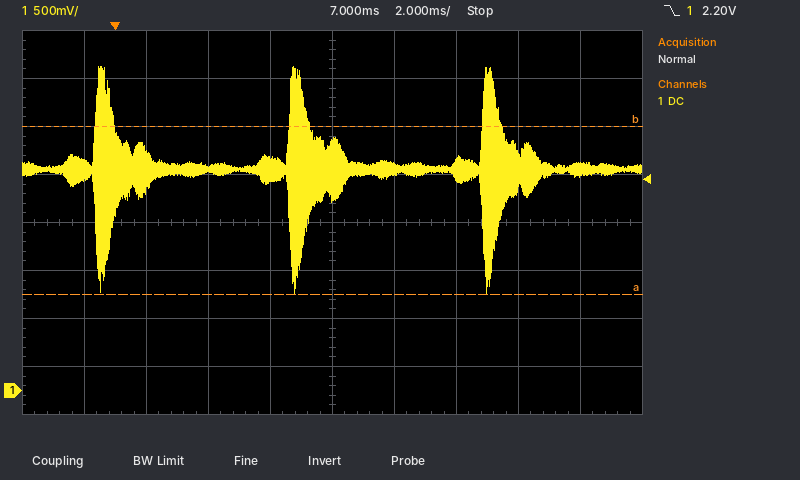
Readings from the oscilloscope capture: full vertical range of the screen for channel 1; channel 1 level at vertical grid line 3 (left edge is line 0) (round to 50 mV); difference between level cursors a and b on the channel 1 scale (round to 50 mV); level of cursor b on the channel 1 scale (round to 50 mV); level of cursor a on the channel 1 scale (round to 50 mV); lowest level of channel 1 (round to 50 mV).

4 V
2.30 V
1.75 V
2.75 V
1.00 V
1.00 V
